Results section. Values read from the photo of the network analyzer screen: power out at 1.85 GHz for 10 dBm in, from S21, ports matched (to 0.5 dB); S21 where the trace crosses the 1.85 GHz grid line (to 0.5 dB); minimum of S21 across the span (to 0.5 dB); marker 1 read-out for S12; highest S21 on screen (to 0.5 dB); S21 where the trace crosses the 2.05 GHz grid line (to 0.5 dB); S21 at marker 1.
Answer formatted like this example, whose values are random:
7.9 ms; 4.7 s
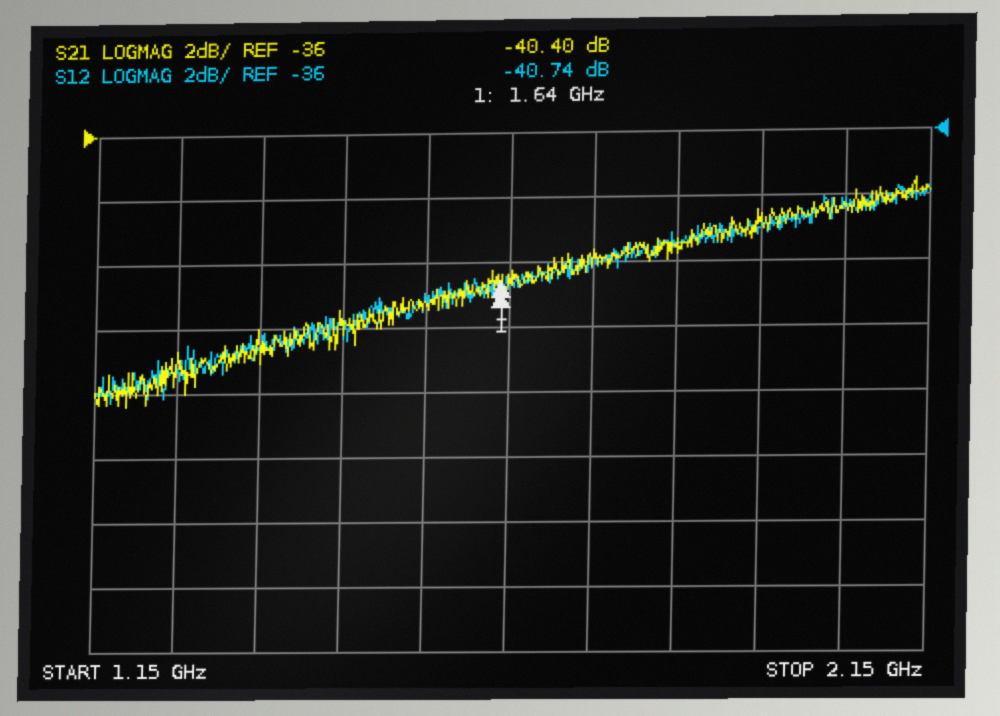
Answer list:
-29.5 dBm; -39.5 dB; -44.5 dB; -40.74 dB; -37.5 dB; -38.5 dB; -40.40 dB
